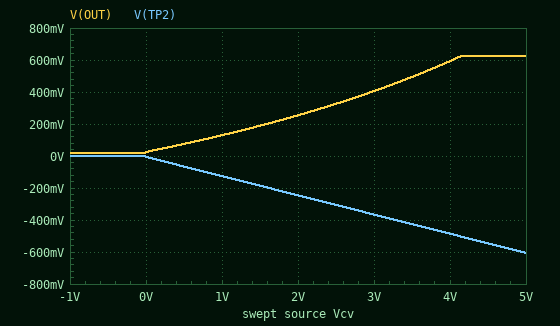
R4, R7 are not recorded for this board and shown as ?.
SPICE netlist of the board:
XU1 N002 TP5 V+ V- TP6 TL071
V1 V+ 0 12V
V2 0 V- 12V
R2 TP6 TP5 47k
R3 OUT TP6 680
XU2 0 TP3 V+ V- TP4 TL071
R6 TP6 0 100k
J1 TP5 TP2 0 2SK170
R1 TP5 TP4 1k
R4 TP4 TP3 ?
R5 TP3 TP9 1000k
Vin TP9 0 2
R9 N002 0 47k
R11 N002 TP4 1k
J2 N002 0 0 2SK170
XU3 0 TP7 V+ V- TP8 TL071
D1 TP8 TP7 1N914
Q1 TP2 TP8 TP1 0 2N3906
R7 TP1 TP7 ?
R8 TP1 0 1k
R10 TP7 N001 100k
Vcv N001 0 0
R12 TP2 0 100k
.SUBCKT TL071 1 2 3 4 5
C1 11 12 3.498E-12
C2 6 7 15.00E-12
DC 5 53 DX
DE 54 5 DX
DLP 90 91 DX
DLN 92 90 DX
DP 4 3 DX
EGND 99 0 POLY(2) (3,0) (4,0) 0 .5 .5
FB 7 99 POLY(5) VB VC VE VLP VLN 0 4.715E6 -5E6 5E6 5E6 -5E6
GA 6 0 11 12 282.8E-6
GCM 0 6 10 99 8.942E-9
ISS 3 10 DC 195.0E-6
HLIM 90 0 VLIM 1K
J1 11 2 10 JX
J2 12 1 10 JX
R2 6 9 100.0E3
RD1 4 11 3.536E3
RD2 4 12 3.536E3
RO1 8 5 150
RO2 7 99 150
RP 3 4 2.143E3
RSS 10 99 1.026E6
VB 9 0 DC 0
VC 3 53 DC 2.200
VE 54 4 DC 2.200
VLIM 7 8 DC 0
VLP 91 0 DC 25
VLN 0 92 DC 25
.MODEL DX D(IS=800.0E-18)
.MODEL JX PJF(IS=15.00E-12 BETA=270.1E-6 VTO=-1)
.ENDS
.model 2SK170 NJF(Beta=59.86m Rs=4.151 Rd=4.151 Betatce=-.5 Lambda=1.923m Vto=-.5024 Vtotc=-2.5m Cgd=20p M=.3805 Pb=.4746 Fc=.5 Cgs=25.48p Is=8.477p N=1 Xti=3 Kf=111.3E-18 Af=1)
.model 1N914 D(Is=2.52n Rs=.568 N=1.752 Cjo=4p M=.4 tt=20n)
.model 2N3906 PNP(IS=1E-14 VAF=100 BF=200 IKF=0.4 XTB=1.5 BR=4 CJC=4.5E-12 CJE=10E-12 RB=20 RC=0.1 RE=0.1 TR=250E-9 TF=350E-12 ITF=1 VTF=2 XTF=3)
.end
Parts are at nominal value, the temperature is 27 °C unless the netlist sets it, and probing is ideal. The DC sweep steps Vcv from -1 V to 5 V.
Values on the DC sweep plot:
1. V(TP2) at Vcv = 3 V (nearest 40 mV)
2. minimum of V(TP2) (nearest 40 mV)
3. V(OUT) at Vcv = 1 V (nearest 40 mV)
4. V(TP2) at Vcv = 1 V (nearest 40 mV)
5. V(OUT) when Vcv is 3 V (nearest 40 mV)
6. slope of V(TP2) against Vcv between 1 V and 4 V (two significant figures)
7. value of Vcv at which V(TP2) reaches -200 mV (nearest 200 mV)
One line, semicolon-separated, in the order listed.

-360 mV; -600 mV; 120 mV; -120 mV; 400 mV; -0.12 V/V; 1.6 V
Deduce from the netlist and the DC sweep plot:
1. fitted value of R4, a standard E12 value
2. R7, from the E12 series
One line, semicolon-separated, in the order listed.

6.8 kΩ; 12 kΩ
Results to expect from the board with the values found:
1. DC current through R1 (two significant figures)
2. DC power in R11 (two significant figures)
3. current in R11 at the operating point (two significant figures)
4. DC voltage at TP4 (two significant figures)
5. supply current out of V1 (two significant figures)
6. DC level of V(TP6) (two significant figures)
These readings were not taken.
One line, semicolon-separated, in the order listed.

13 µA; 180 nW; 13 µA; -14 mV; 34 mA; 21 mV
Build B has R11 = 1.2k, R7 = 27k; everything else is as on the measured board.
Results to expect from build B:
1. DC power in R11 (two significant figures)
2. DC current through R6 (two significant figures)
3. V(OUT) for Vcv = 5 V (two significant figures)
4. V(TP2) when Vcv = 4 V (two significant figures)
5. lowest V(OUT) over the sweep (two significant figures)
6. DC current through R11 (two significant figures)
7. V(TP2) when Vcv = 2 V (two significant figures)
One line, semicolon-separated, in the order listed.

150 nW; 1.2 µA; 630 mV; -1.1 V; 120 mV; 11 µA; -550 mV
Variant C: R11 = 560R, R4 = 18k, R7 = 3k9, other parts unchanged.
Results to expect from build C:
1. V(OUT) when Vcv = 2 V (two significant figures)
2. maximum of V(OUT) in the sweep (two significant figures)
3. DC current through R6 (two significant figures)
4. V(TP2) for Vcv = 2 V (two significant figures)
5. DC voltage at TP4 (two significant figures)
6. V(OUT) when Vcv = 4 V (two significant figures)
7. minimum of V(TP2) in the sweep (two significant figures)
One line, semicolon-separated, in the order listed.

-910 mV; -370 mV; 12 µA; -84 mV; -36 mV; -560 mV; -200 mV
